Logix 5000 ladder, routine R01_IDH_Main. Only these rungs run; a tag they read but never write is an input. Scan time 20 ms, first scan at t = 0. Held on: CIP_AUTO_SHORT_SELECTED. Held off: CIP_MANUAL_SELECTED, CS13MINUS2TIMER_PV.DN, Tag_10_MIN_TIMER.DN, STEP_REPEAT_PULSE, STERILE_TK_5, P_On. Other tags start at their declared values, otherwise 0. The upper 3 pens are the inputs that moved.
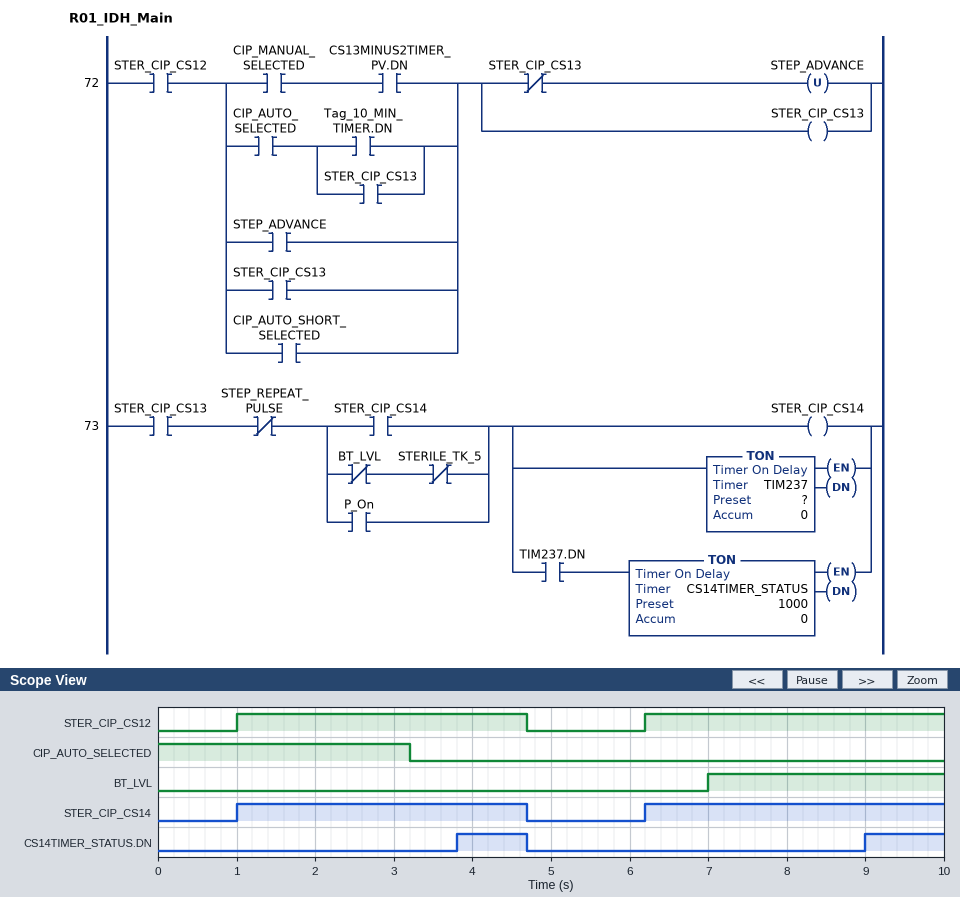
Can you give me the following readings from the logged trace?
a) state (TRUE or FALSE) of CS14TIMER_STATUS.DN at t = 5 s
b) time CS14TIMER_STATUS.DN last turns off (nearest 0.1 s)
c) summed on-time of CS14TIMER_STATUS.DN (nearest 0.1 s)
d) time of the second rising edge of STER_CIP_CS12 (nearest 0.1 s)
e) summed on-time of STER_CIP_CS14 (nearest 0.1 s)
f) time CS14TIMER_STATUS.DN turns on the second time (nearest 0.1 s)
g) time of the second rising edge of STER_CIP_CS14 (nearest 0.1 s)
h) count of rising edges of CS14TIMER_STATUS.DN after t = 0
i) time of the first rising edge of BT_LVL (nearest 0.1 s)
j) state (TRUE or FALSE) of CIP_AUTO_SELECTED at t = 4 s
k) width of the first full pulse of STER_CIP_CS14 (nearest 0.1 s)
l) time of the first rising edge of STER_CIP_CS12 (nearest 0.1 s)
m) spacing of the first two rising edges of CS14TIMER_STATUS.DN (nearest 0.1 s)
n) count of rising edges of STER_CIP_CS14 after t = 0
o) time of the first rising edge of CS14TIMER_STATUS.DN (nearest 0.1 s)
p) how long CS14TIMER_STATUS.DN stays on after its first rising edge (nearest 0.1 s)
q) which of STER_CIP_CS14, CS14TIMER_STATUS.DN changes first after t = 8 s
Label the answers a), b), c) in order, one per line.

a) FALSE
b) 4.7 s
c) 1.9 s
d) 6.2 s
e) 7.5 s
f) 9.0 s
g) 6.2 s
h) 2
i) 7.0 s
j) FALSE
k) 3.7 s
l) 1.0 s
m) 5.2 s
n) 2
o) 3.8 s
p) 0.9 s
q) CS14TIMER_STATUS.DN
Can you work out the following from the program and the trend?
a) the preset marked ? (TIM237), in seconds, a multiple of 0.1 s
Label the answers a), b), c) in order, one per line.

a) 1.8 s
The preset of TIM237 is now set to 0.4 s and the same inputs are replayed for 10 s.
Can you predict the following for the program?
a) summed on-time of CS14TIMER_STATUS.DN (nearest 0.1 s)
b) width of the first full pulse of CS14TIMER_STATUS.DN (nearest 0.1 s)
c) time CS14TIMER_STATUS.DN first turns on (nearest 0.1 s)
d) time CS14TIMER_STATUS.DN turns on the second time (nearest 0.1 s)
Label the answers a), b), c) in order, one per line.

a) 4.7 s
b) 2.3 s
c) 2.4 s
d) 7.6 s
